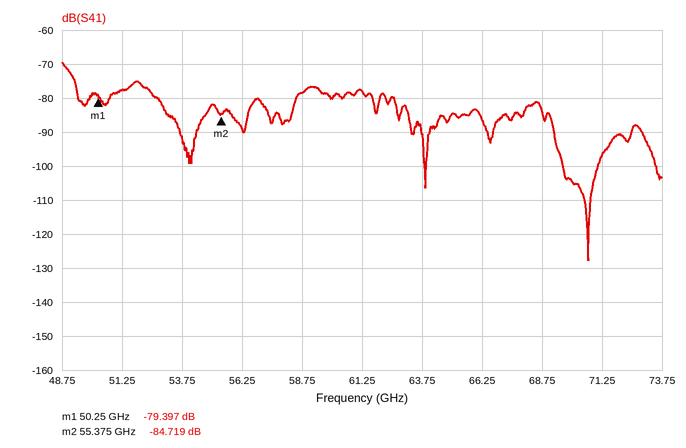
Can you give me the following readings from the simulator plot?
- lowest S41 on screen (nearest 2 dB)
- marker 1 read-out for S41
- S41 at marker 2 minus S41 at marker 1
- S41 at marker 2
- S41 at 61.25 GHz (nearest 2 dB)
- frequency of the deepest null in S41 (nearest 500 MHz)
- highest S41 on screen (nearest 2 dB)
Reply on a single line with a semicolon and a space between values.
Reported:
-128 dB; -79.397 dB; -5.322 dB; -84.719 dB; -78 dB; 70.5 GHz; -70 dB
